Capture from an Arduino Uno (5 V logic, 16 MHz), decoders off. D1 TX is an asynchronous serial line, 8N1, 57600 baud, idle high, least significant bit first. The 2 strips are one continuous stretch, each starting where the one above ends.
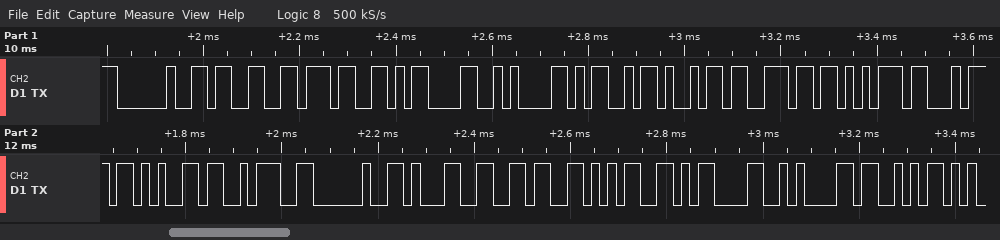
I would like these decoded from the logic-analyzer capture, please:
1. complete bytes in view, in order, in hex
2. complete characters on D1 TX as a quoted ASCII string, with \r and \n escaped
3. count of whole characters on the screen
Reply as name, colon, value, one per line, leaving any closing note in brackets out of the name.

complete bytes in view, in order, in hex: 20 33 37 0D 0A 4D 69 6E 75 74 65 3A 20 31 36 35 0D 0A 53
complete characters on D1 TX as a quoted ASCII string, with \r and \n escaped: " 37\r\nMinute: 165\r\nS"
count of whole characters on the screen: 19
